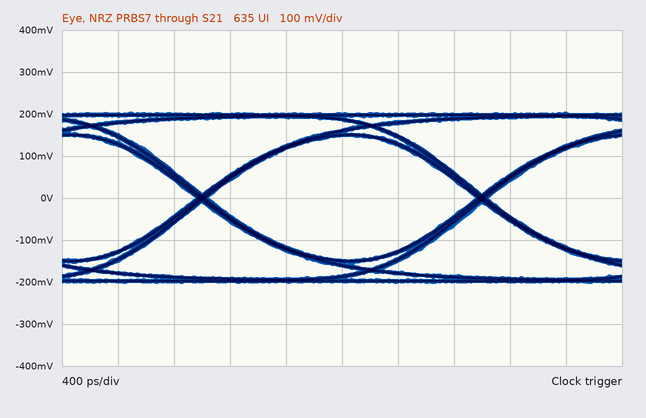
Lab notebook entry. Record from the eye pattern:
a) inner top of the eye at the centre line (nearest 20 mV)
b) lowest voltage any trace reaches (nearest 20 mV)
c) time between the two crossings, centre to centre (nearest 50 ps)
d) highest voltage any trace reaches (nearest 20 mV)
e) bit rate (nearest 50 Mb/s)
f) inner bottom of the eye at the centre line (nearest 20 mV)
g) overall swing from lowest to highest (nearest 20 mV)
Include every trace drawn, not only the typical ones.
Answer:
140 mV
-200 mV
2.00 ns
200 mV
500 Mb/s
-140 mV
400 mV
